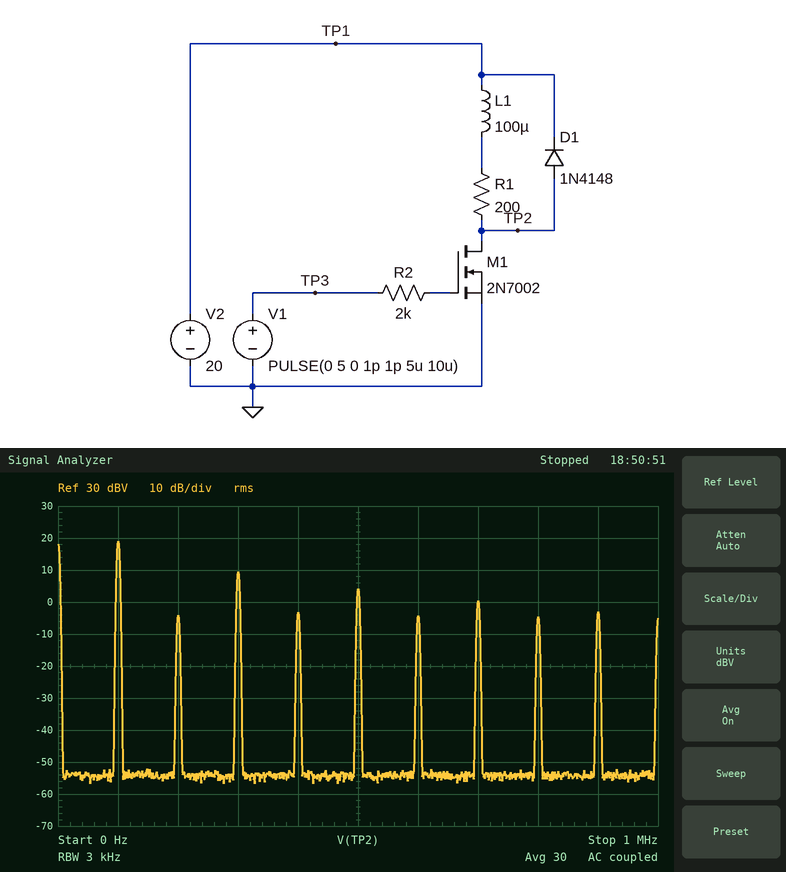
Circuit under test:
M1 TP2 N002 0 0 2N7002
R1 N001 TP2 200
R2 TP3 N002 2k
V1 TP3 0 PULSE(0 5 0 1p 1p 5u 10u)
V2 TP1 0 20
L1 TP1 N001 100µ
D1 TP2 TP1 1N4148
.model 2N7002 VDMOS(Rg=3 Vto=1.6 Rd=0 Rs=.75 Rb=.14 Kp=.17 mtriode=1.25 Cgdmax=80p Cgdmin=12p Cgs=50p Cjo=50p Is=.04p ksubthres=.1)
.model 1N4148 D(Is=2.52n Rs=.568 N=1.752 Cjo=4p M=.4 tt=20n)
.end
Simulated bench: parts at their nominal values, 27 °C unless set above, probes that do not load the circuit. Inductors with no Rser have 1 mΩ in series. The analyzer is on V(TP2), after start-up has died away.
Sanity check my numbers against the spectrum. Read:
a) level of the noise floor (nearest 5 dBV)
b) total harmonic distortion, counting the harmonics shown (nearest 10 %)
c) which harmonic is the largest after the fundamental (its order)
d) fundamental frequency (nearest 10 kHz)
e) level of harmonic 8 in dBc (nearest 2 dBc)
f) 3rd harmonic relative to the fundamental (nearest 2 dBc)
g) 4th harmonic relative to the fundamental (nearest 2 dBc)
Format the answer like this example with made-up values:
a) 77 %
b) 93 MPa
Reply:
a) -55 dBV
b) 40 %
c) 3
d) 100 kHz
e) -24 dBc
f) -10 dBc
g) -22 dBc
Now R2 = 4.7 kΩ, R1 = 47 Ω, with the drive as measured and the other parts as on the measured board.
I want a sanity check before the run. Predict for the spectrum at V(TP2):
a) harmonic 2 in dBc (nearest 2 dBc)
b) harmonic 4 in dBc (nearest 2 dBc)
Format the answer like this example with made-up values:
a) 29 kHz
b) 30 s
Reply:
a) -30 dBc
b) -28 dBc
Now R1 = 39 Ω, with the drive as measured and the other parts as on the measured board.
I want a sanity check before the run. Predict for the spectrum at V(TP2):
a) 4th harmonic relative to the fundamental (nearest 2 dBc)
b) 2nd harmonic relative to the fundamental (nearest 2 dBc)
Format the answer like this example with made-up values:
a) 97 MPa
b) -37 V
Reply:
a) -48 dBc
b) -42 dBc
